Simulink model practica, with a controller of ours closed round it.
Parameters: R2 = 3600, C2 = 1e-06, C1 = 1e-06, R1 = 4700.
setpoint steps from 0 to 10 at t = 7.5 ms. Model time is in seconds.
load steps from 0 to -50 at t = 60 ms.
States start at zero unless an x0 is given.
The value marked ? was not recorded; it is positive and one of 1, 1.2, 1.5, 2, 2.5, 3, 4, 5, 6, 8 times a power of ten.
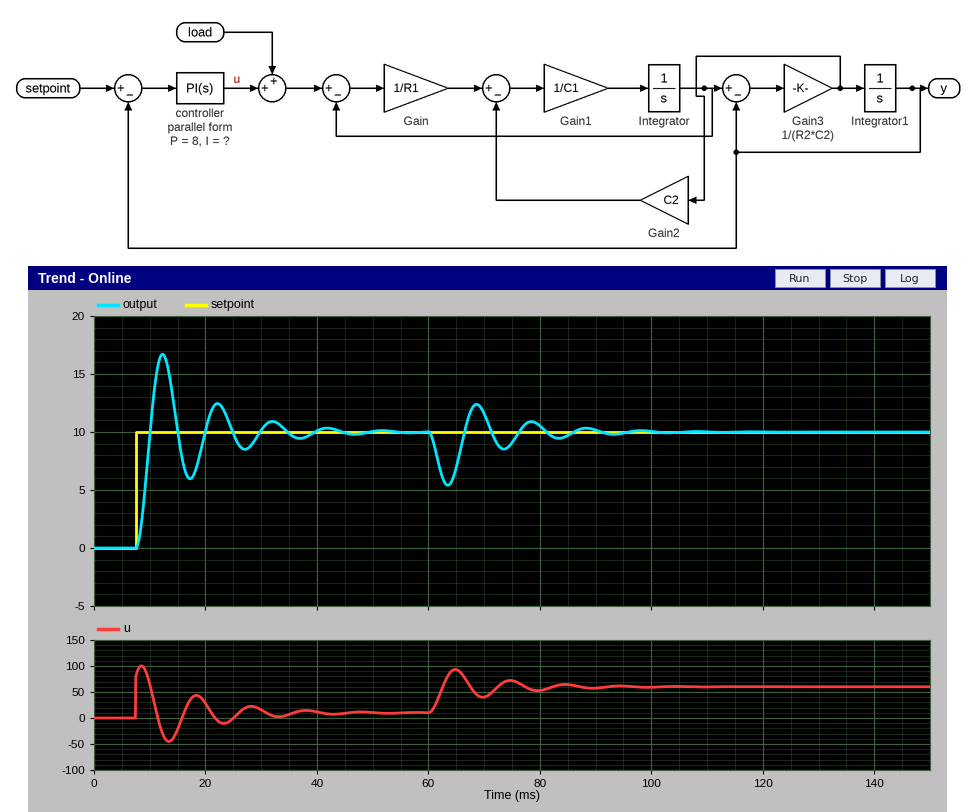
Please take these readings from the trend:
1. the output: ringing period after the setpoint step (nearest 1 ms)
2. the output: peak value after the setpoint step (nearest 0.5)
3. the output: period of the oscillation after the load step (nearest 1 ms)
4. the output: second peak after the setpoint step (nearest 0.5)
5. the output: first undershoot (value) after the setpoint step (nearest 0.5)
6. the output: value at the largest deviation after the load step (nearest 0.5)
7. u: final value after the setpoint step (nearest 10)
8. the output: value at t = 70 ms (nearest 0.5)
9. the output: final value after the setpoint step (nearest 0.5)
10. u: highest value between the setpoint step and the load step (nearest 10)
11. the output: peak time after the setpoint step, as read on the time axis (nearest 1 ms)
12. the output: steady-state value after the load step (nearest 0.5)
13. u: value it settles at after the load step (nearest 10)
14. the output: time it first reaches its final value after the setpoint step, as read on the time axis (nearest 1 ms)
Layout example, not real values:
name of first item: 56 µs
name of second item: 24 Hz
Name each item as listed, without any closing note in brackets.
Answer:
the output: ringing period after the setpoint step: 10 ms
the output: peak value after the setpoint step: 16.5
the output: period of the oscillation after the load step: 10 ms
the output: second peak after the setpoint step: 12.5
the output: first undershoot (value) after the setpoint step: 6.0
the output: value at the largest deviation after the load step: 5.5
u: final value after the setpoint step: 10
the output: value at t = 70 ms: 11.5
the output: final value after the setpoint step: 10.0
u: highest value between the setpoint step and the load step: 100
the output: peak time after the setpoint step, as read on the time axis: 12 ms
the output: steady-state value after the load step: 10.0
u: value it settles at after the load step: 60
the output: time it first reaches its final value after the setpoint step, as read on the time axis: 10 ms
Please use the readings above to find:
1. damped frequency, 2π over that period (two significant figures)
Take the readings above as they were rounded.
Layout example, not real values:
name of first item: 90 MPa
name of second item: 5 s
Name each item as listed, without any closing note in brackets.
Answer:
damped frequency, 2π over that period: 0.63 rad/ms
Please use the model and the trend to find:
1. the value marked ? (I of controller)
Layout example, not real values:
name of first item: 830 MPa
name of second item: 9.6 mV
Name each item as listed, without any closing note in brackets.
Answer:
the value marked ?: 4000
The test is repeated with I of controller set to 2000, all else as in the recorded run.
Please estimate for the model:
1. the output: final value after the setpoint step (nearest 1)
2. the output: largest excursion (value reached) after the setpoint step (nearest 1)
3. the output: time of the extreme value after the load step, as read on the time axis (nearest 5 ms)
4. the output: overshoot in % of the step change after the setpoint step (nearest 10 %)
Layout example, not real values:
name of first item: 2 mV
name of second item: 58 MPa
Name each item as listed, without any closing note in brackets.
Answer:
the output: final value after the setpoint step: 10
the output: largest excursion (value reached) after the setpoint step: 14
the output: time of the extreme value after the load step, as read on the time axis: 65 ms
the output: overshoot in % of the step change after the setpoint step: 40 %
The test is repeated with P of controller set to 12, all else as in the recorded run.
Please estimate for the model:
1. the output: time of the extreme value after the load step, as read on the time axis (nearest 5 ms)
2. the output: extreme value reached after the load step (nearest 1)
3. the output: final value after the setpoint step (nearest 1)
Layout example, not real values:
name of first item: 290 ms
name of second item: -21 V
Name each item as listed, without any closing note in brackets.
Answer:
the output: time of the extreme value after the load step, as read on the time axis: 65 ms
the output: extreme value reached after the load step: 6
the output: final value after the setpoint step: 10
